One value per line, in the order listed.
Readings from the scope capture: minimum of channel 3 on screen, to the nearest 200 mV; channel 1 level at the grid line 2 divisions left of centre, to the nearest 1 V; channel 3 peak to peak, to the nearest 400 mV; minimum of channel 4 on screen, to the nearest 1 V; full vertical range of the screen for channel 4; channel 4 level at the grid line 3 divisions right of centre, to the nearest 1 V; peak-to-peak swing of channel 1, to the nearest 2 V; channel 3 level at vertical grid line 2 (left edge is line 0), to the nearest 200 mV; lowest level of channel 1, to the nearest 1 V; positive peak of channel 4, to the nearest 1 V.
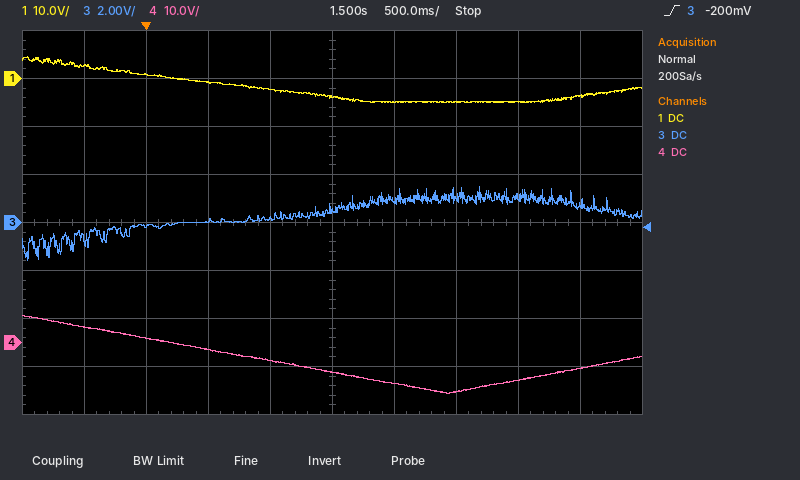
-1.6 V
-1 V
3.2 V
-11 V
80 V
-8 V
10 V
-200 mV
-5 V
6 V
